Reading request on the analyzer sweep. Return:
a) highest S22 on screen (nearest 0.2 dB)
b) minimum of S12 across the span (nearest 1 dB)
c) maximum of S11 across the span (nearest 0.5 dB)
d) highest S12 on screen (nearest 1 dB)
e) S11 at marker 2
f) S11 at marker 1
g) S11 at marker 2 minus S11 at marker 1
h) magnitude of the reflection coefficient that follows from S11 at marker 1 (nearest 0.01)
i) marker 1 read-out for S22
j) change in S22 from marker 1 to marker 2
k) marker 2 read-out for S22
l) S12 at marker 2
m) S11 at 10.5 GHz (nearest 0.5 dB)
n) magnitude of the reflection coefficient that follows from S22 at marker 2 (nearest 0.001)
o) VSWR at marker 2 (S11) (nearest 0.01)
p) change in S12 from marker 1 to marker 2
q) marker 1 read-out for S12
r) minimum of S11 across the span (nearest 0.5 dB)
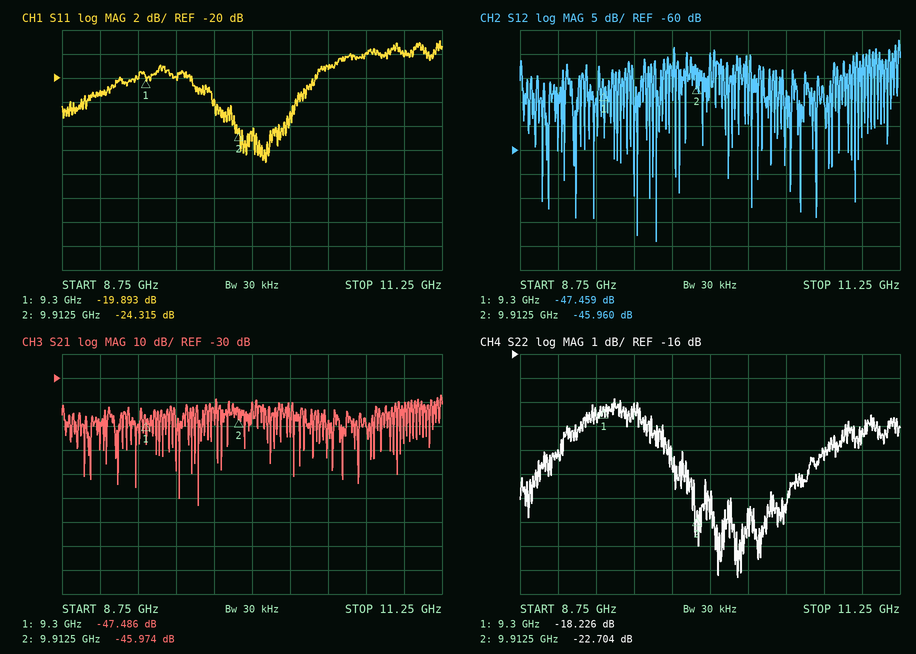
-17.8 dB
-79 dB
-17.0 dB
-37 dB
-24.315 dB
-19.893 dB
-4.422 dB
0.10
-18.226 dB
-4.478 dB
-22.704 dB
-45.960 dB
-19.0 dB
0.073
1.13
1.499 dB
-47.459 dB
-27.0 dB
